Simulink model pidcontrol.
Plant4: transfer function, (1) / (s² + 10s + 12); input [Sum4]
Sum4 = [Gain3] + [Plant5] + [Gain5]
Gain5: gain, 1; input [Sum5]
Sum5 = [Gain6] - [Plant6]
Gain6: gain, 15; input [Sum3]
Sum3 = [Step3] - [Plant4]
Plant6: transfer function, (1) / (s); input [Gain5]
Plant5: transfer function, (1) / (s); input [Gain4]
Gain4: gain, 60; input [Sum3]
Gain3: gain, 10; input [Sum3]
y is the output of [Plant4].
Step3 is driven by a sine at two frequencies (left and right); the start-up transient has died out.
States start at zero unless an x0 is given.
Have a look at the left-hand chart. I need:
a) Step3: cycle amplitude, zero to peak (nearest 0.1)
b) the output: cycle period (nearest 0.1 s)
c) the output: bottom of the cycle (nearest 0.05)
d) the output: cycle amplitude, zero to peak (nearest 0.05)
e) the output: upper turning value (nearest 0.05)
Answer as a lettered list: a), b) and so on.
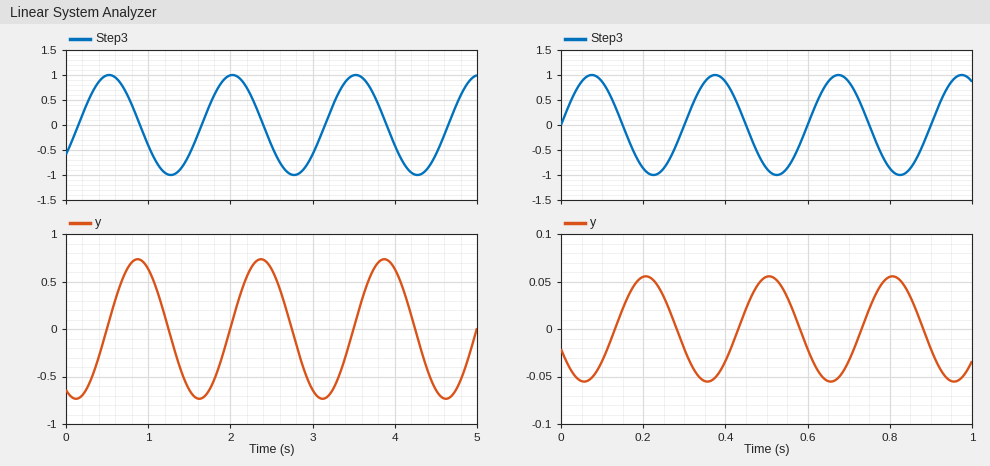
a) 1.0
b) 1.5 s
c) -0.75
d) 0.75
e) 0.75
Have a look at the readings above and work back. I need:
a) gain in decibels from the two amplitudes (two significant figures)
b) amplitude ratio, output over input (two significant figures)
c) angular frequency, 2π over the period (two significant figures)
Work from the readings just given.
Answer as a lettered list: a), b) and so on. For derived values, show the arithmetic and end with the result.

a) 20 log10(0.75 / 1) = -2.5 dB
b) 0.75 / 1 = 0.75
c) 2π / 1.5 = 4.2 rad/s
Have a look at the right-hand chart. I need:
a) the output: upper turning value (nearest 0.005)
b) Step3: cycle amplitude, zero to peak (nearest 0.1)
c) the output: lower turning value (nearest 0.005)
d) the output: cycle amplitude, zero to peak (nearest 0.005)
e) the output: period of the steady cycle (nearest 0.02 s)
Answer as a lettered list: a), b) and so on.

a) 0.055
b) 1.0
c) -0.055
d) 0.055
e) 0.30 s
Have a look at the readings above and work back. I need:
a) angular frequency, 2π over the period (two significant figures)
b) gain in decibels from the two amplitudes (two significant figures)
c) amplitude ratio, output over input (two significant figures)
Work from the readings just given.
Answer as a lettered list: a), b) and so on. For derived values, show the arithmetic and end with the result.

a) 2π / 0.3 = 21 rad/s
b) 20 log10(0.055 / 1) = -25 dB
c) 0.055 / 1 = 0.055
